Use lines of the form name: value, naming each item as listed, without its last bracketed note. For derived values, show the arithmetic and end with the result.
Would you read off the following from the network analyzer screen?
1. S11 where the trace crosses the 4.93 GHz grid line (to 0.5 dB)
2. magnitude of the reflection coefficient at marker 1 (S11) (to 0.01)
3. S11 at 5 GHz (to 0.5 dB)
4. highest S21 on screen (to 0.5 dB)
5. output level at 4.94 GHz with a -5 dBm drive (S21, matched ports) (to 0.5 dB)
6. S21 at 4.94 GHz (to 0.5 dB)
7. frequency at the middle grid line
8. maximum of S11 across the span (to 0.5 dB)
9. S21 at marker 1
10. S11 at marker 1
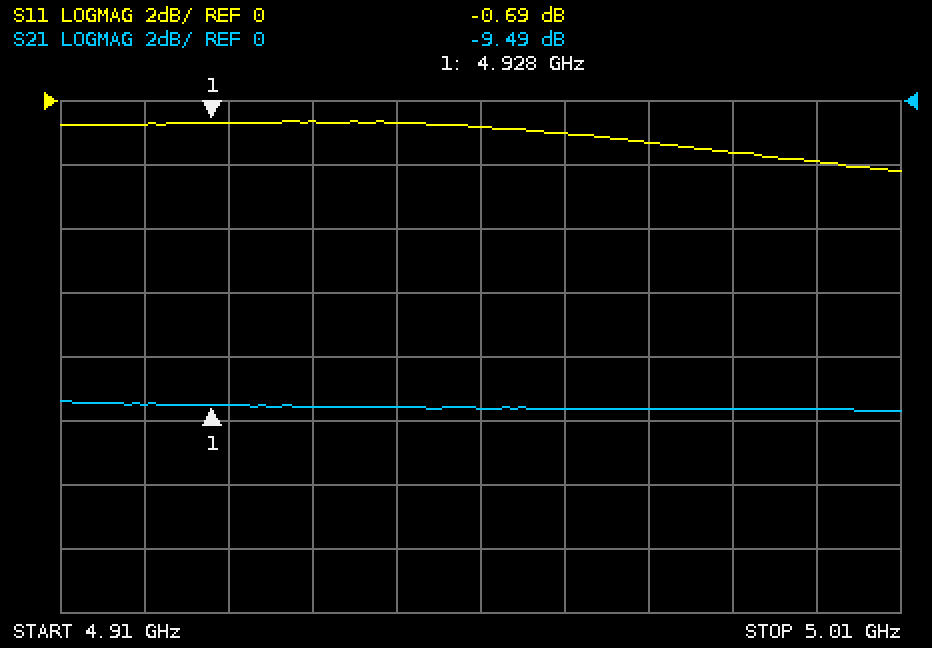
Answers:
S11 where the trace crosses the 4.93 GHz grid line: -0.5 dB
magnitude of the reflection coefficient at marker 1 (S11): 10^(-0.69/20) ≈ 0.92
S11 at 5 GHz: -2.0 dB
highest S21 on screen: -9.5 dB
output level at 4.94 GHz with a -5 dBm drive (S21, matched ports): -5 dBm + (-9.5 dB) = -14.5 dBm
S21 at 4.94 GHz: -9.5 dB
frequency at the middle grid line: 4.96 GHz
maximum of S11 across the span: -0.5 dB
S21 at marker 1: -9.49 dB
S11 at marker 1: -0.69 dB
